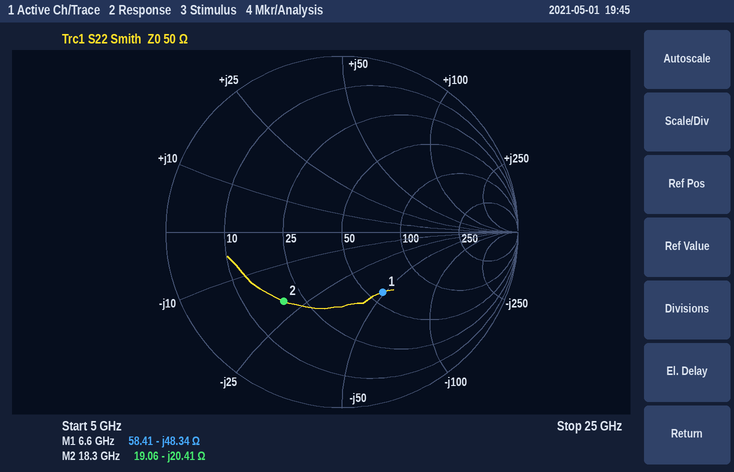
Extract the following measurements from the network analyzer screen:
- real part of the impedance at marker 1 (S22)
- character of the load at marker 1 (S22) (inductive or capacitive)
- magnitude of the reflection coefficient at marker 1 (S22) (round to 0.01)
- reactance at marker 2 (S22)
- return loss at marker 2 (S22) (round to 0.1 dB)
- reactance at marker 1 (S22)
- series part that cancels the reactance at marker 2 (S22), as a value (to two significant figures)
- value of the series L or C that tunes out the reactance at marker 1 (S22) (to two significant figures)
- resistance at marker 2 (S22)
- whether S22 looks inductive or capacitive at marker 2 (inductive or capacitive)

58.41 Ω
capacitive
0.41
-20.41 Ω
5.8 dB
-48.34 Ω
180 pH
1.2 nH
19.06 Ω
capacitive
